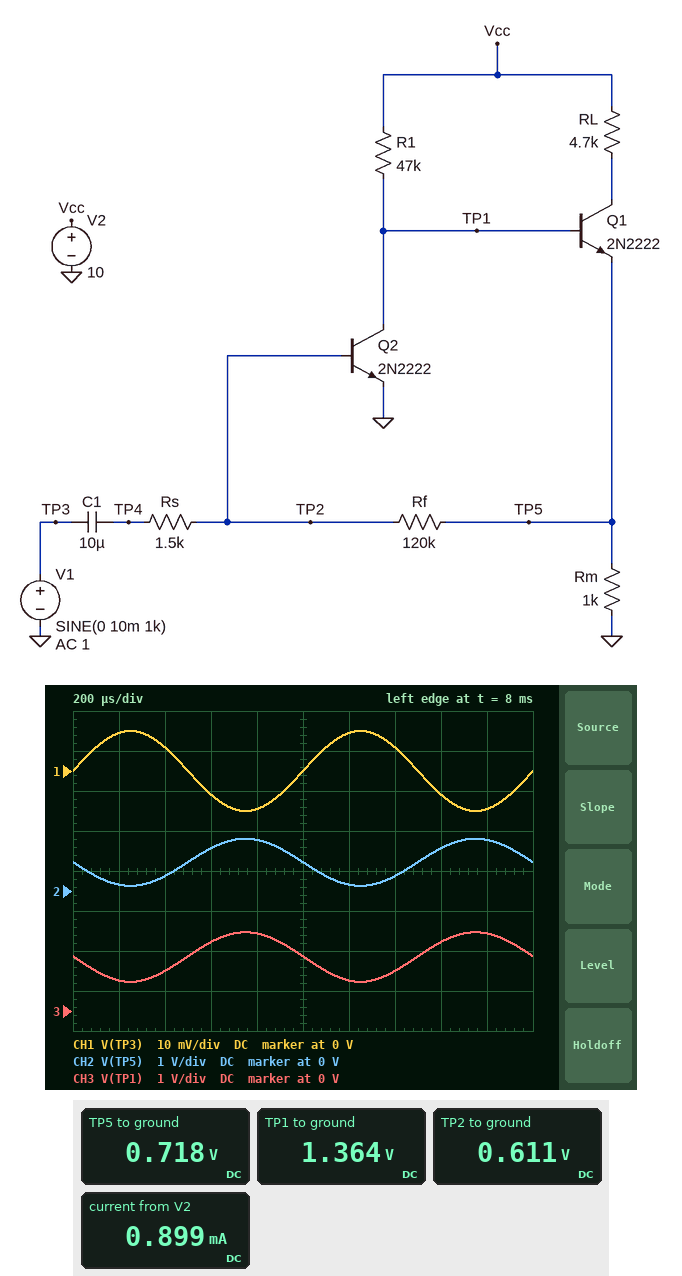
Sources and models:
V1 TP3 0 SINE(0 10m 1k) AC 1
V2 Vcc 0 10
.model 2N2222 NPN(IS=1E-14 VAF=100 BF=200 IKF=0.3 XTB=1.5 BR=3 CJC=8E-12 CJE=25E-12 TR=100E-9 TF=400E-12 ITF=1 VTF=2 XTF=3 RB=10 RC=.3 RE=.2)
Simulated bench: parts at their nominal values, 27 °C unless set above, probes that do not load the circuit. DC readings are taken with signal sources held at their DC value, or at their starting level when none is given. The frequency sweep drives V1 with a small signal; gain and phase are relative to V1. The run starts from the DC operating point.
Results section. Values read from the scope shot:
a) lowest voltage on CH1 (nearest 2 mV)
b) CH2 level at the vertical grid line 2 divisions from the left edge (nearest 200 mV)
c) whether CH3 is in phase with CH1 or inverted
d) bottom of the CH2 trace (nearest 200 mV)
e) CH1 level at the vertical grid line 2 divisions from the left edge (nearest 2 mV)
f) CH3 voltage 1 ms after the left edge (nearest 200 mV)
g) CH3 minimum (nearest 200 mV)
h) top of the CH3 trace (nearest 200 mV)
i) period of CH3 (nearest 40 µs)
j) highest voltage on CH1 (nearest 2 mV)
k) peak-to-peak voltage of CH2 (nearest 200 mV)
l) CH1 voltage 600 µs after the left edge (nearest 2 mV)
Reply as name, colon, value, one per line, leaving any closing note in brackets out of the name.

lowest voltage on CH1: -10 mV
CH2 level at the vertical grid line 2 divisions from the left edge: 400 mV
whether CH3 is in phase with CH1 or inverted: inverted
bottom of the CH2 trace: 200 mV
CH1 level at the vertical grid line 2 divisions from the left edge: 6 mV
CH3 voltage 1 ms after the left edge: 1.4 V
CH3 minimum: 800 mV
top of the CH3 trace: 2.0 V
period of CH3: 1.00 ms
highest voltage on CH1: 10 mV
peak-to-peak voltage of CH2: 1.2 V
CH1 voltage 600 µs after the left edge: -6 mV
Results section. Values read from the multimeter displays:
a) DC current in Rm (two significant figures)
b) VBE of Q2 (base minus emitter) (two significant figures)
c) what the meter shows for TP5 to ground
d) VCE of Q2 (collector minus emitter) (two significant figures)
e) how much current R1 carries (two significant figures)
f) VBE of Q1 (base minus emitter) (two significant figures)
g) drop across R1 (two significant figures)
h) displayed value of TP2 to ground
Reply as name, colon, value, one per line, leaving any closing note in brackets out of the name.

DC current in Rm: 720 µA
VBE of Q2 (base minus emitter): 610 mV
what the meter shows for TP5 to ground: 0.718 V
VCE of Q2 (collector minus emitter): 1.4 V
how much current R1 carries: 180 µA
VBE of Q1 (base minus emitter): 650 mV
drop across R1: 8.6 V
displayed value of TP2 to ground: 0.611 V
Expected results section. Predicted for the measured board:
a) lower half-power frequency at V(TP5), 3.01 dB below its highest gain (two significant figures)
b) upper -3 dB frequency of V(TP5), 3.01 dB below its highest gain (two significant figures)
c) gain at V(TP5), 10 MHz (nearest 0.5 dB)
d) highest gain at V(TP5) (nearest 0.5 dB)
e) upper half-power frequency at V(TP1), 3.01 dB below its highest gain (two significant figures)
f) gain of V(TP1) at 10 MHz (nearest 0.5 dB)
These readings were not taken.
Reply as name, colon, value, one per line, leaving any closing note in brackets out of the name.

lower half-power frequency at V(TP5), 3.01 dB below its highest gain: 8.0 Hz
upper -3 dB frequency of V(TP5), 3.01 dB below its highest gain: 180 kHz
gain at V(TP5), 10 MHz: -3.0 dB
highest gain at V(TP5): 35.5 dB
upper half-power frequency at V(TP1), 3.01 dB below its highest gain: 180 kHz
gain of V(TP1) at 10 MHz: -2.5 dB
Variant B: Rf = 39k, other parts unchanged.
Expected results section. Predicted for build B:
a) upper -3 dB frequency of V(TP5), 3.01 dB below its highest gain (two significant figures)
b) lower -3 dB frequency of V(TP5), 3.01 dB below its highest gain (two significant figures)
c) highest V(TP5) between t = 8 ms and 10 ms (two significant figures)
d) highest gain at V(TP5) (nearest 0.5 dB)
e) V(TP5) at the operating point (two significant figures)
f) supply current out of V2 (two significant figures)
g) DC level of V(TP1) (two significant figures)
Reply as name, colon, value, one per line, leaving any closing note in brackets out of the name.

upper -3 dB frequency of V(TP5), 3.01 dB below its highest gain: 460 kHz
lower -3 dB frequency of V(TP5), 3.01 dB below its highest gain: 9.6 Hz
highest V(TP5) between t = 8 ms and 10 ms: 880 mV
highest gain at V(TP5): 27.5 dB
V(TP5) at the operating point: 650 mV
supply current out of V2: 830 µA
DC level of V(TP1): 1.3 V
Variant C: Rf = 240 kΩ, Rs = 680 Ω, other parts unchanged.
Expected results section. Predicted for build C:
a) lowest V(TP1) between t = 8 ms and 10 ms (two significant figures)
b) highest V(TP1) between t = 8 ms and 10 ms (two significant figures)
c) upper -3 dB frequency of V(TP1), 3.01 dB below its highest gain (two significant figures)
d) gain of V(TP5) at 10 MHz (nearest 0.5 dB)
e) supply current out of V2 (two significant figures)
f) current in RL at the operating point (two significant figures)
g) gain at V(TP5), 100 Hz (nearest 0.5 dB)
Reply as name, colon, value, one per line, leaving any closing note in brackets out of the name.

lowest V(TP1) between t = 8 ms and 10 ms: 92 mV
highest V(TP1) between t = 8 ms and 10 ms: 2.4 V
upper -3 dB frequency of V(TP1), 3.01 dB below its highest gain: 120 kHz
gain of V(TP5) at 10 MHz: 3.0 dB
supply current out of V2: 1.0 mA
current in RL at the operating point: 820 µA
gain at V(TP5), 100 Hz: 43.0 dB
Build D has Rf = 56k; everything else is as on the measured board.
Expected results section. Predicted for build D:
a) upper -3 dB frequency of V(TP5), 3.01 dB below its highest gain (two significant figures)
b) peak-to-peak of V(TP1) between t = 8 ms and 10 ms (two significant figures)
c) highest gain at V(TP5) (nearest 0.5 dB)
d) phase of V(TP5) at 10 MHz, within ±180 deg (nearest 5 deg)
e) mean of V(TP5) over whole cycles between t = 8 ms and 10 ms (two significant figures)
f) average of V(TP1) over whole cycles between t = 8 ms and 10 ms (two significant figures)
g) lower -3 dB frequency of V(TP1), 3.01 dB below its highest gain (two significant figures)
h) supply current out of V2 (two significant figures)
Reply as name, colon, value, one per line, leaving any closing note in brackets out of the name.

upper -3 dB frequency of V(TP5), 3.01 dB below its highest gain: 340 kHz
peak-to-peak of V(TP1) between t = 8 ms and 10 ms: 670 mV
highest gain at V(TP5): 30.0 dB
phase of V(TP5) at 10 MHz, within ±180 deg: 65 deg
mean of V(TP5) over whole cycles between t = 8 ms and 10 ms: 660 mV
average of V(TP1) over whole cycles between t = 8 ms and 10 ms: 1.3 V
lower -3 dB frequency of V(TP1), 3.01 dB below its highest gain: 9.2 Hz
supply current out of V2: 840 µA
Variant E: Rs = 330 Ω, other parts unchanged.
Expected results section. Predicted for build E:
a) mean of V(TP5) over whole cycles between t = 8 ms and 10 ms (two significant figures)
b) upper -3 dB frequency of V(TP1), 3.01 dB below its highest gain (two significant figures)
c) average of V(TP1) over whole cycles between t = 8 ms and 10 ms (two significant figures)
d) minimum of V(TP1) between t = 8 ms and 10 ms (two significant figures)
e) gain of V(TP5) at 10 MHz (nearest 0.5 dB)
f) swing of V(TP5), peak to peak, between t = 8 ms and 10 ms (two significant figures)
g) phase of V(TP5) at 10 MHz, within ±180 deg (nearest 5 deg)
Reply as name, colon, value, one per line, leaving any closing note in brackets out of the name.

mean of V(TP5) over whole cycles between t = 8 ms and 10 ms: 810 mV
upper -3 dB frequency of V(TP1), 3.01 dB below its highest gain: 160 kHz
average of V(TP1) over whole cycles between t = 8 ms and 10 ms: 1.3 V
minimum of V(TP1) between t = 8 ms and 10 ms: 75 mV
gain of V(TP5) at 10 MHz: 7.5 dB
swing of V(TP5), peak to peak, between t = 8 ms and 10 ms: 1.7 V
phase of V(TP5) at 10 MHz, within ±180 deg: 85 deg
